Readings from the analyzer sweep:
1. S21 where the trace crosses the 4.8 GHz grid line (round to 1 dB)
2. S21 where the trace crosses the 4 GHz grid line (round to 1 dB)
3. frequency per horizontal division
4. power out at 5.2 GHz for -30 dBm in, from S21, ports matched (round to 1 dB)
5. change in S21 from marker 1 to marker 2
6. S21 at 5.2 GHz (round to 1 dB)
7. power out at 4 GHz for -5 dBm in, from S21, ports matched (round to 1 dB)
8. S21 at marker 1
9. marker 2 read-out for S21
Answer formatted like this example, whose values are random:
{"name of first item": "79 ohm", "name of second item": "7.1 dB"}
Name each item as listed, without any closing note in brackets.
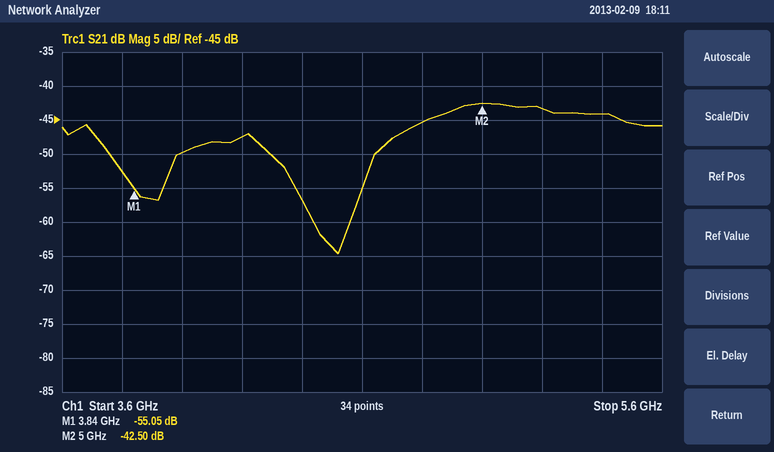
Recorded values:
{"S21 where the trace crosses the 4.8 GHz grid line": "-45 dB", "S21 where the trace crosses the 4 GHz grid line": "-50 dB", "frequency per horizontal division": "200 MHz", "power out at 5.2 GHz for -30 dBm in, from S21, ports matched": "-73 dBm", "change in S21 from marker 1 to marker 2": "12.55 dB", "S21 at 5.2 GHz": "-43 dB", "power out at 4 GHz for -5 dBm in, from S21, ports matched": "-55 dBm", "S21 at marker 1": "-55.05 dB", "marker 2 read-out for S21": "-42.50 dB"}
